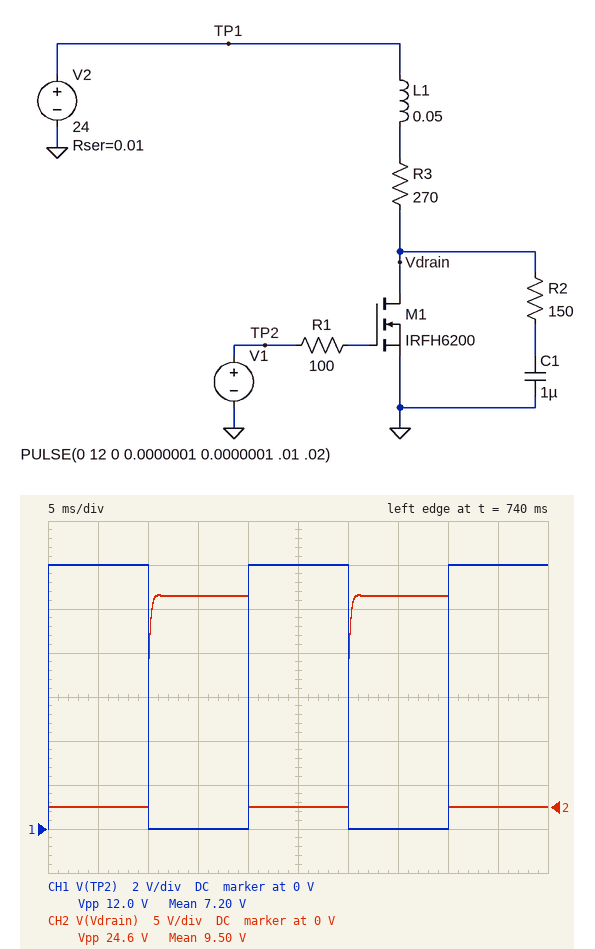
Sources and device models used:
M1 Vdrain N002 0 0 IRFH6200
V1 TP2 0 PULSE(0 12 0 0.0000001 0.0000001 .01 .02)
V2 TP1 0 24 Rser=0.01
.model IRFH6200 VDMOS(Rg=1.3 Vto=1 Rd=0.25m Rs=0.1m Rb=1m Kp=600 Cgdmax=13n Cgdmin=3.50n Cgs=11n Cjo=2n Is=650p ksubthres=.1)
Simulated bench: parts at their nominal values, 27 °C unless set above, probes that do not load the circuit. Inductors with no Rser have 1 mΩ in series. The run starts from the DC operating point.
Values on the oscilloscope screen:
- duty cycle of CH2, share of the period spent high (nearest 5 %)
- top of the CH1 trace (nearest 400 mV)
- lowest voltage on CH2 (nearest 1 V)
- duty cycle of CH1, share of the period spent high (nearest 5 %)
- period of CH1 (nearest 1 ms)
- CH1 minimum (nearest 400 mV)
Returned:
50 %
12.0 V
0 V
50 %
20 ms
0 V
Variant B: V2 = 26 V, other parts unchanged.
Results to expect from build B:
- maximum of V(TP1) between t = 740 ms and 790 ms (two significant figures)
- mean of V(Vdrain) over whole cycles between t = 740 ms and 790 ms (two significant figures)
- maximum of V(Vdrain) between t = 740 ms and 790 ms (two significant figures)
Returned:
26 V
13 V
27 V
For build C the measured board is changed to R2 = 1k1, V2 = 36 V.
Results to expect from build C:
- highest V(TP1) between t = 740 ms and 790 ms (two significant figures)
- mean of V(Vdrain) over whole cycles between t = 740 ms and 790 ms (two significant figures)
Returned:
36 V
18 V
